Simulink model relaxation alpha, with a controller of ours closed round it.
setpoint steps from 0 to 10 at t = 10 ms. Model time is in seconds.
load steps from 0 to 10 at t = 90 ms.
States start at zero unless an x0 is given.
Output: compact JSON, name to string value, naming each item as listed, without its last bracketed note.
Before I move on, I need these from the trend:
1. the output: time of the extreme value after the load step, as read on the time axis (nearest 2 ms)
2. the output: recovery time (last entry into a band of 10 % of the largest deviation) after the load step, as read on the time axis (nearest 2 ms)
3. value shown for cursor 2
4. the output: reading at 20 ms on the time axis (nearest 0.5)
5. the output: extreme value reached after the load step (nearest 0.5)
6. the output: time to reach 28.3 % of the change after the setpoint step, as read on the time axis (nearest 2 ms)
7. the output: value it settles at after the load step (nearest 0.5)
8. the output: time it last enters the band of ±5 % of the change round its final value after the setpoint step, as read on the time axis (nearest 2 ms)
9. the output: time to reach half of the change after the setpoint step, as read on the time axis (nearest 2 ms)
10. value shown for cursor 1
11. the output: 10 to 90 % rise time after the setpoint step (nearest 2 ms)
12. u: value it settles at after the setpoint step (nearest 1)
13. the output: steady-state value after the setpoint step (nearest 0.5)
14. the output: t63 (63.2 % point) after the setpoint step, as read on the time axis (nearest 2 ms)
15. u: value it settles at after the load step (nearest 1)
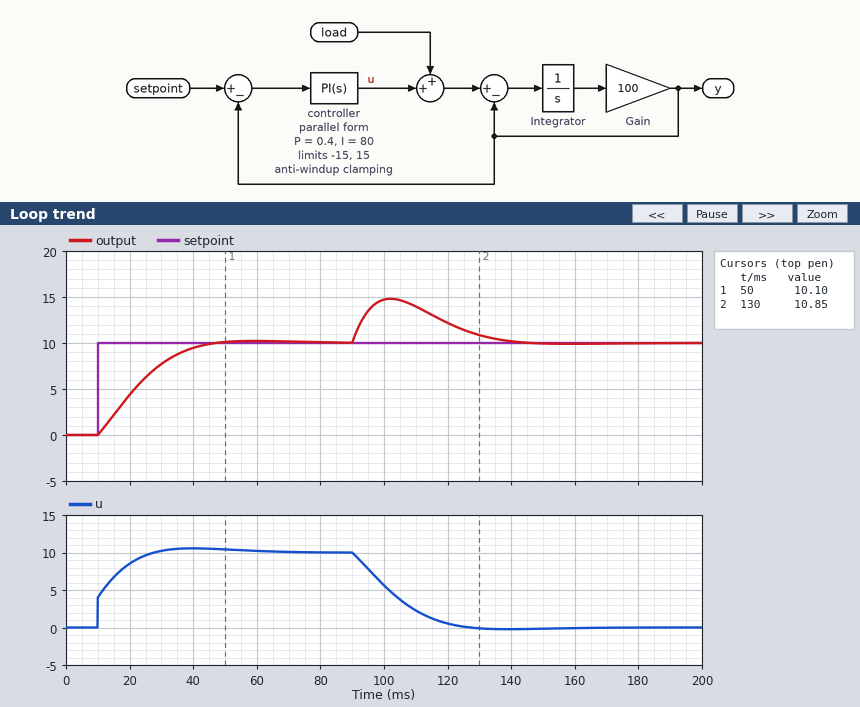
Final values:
{"the output: time of the extreme value after the load step, as read on the time axis": "102 ms", "the output: recovery time (last entry into a band of 10 % of the largest deviation) after the load step, as read on the time axis": "134 ms", "value shown for cursor 2": "10.85", "the output: reading at 20 ms on the time axis": "4.5", "the output: extreme value reached after the load step": "15.0", "the output: time to reach 28.3 % of the change after the setpoint step, as read on the time axis": "16 ms", "the output: value it settles at after the load step": "10.0", "the output: time it last enters the band of ±5 % of the change round its final value after the setpoint step, as read on the time axis": "40 ms", "the output: time to reach half of the change after the setpoint step, as read on the time axis": "22 ms", "value shown for cursor 1": "10.10", "the output: 10 to 90 % rise time after the setpoint step": "24 ms", "u: value it settles at after the setpoint step": "10", "the output: steady-state value after the setpoint step": "10.0", "the output: t63 (63.2 % point) after the setpoint step, as read on the time axis": "26 ms", "u: value it settles at after the load step": "0"}
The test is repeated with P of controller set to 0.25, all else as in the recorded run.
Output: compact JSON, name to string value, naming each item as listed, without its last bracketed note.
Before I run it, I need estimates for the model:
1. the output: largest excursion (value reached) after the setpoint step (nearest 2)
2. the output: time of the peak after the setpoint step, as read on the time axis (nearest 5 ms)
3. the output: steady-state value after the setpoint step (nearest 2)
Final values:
{"the output: largest excursion (value reached) after the setpoint step": "10", "the output: time of the peak after the setpoint step, as read on the time axis": "55 ms", "the output: steady-state value after the setpoint step": "10"}
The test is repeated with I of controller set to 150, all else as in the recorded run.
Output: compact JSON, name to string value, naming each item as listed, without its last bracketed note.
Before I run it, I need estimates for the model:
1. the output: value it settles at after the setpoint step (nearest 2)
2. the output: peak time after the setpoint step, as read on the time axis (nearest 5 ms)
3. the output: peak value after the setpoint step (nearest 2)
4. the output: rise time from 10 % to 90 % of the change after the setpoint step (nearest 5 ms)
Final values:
{"the output: value it settles at after the setpoint step": "10", "the output: peak time after the setpoint step, as read on the time axis": "40 ms", "the output: peak value after the setpoint step": "12", "the output: rise time from 10 % to 90 % of the change after the setpoint step": "15 ms"}
